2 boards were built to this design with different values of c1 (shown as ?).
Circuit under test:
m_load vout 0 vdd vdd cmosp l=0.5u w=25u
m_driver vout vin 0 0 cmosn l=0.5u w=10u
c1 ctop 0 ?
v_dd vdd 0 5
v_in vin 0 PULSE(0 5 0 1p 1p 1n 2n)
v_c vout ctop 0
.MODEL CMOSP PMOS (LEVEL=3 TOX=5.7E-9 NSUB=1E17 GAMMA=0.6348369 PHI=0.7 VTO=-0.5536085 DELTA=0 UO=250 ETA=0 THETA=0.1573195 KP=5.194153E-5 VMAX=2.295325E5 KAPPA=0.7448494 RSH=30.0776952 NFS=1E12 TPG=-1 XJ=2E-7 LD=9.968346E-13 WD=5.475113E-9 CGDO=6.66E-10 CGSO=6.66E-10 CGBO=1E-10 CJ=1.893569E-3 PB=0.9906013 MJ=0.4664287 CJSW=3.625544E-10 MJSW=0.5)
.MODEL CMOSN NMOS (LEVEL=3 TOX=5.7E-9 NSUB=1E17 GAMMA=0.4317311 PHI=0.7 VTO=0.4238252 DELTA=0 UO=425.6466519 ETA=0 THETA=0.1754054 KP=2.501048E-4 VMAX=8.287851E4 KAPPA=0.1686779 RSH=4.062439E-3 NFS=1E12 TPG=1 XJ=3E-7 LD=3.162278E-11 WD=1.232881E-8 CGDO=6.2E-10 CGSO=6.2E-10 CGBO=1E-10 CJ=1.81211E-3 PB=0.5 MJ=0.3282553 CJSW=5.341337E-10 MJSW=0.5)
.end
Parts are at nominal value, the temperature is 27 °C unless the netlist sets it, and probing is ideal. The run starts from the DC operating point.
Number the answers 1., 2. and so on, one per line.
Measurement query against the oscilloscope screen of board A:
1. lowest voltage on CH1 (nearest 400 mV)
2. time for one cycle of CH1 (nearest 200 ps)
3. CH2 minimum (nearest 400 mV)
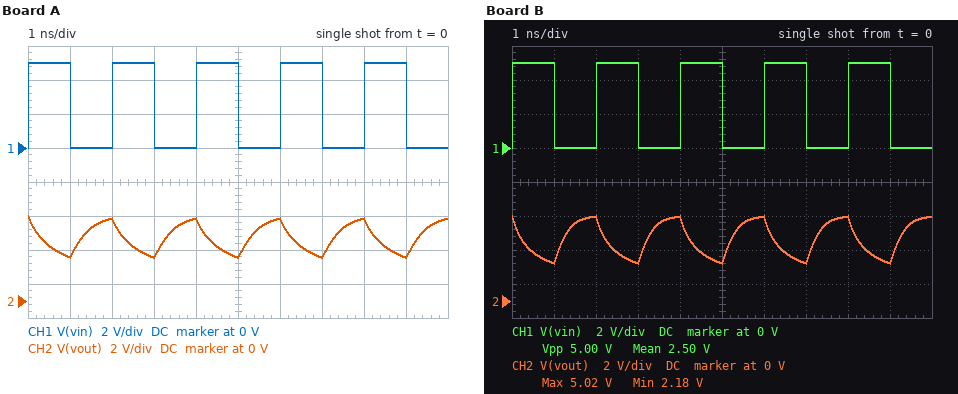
1. 0 V
2. 2.0 ns
3. 2.4 V
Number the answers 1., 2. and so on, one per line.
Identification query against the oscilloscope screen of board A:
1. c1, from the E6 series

1. 1.5 pF
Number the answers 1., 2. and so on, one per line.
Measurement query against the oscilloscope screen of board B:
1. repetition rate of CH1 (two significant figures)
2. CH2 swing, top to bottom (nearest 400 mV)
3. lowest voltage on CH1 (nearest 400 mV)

1. 500 MHz
2. 2.8 V
3. 0 V
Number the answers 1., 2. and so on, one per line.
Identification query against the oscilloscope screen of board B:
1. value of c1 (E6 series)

1. 1 pF
